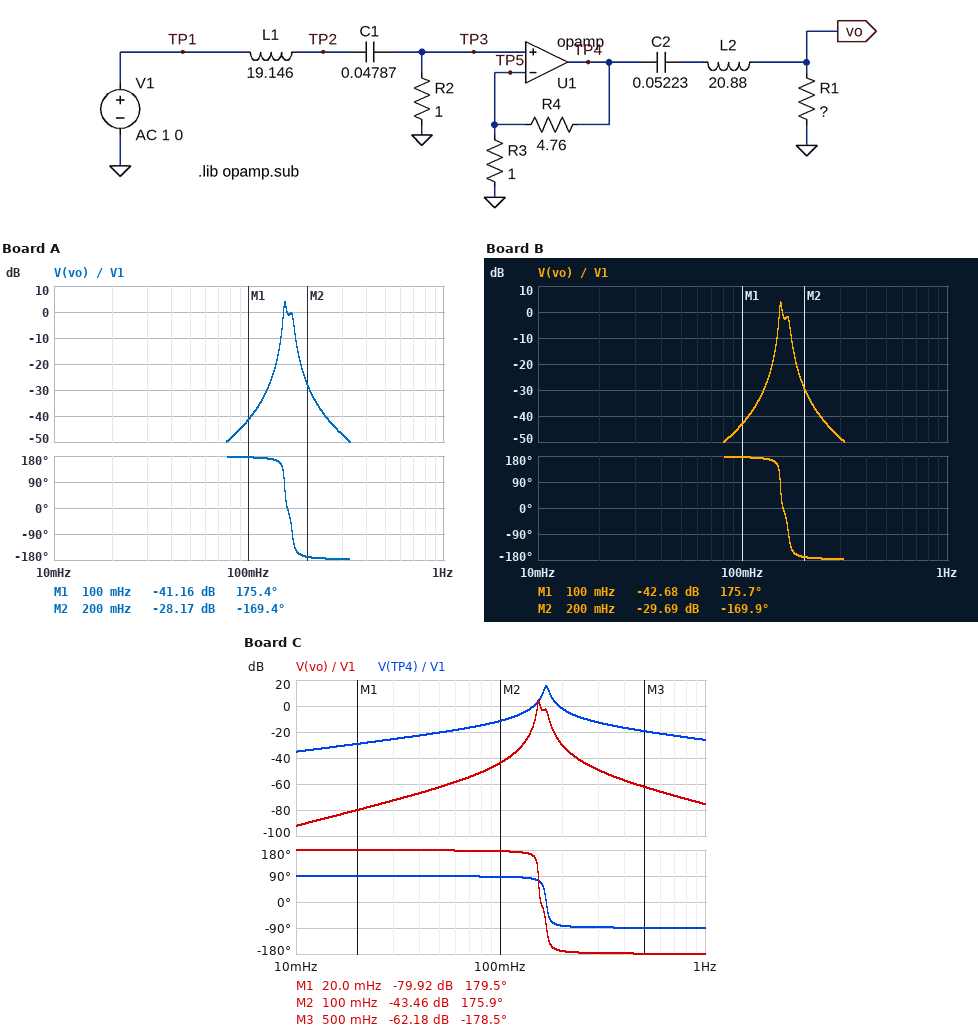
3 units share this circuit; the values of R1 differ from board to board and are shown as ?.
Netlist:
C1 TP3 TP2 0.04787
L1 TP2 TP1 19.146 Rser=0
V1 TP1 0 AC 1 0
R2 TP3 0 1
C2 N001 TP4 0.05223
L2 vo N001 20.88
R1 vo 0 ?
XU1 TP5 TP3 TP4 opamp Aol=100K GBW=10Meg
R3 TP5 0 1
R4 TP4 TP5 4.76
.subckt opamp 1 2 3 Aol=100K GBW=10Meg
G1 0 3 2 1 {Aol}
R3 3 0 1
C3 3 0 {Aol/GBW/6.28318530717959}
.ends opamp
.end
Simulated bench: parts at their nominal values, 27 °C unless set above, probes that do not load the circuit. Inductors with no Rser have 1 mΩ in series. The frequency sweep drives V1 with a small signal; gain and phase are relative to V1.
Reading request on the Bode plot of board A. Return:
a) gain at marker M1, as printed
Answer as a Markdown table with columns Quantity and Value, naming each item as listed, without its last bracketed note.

| Quantity | Value |
|---|---|
| gain at marker M1, as printed | -41.16 dB |
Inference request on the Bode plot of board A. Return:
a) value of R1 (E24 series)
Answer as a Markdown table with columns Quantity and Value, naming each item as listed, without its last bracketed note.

| Quantity | Value |
|---|---|
| value of R1 | 0.56 Ω |
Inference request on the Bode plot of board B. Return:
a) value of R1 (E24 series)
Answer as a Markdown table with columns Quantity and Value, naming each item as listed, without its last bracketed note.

| Quantity | Value |
|---|---|
| value of R1 | 0.47 Ω |
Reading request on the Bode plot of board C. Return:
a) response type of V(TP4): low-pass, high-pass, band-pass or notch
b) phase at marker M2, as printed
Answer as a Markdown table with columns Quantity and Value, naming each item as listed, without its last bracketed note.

| Quantity | Value |
|---|---|
| response type of V(TP4): low-pass, high-pass, band-pass or notch | band-pass |
| phase at marker M2, as printed | 175.9 deg |
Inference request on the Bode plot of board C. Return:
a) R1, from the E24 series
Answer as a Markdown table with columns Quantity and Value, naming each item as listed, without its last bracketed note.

| Quantity | Value |
|---|---|
| R1, from the E24 series | 0.43 Ω |
